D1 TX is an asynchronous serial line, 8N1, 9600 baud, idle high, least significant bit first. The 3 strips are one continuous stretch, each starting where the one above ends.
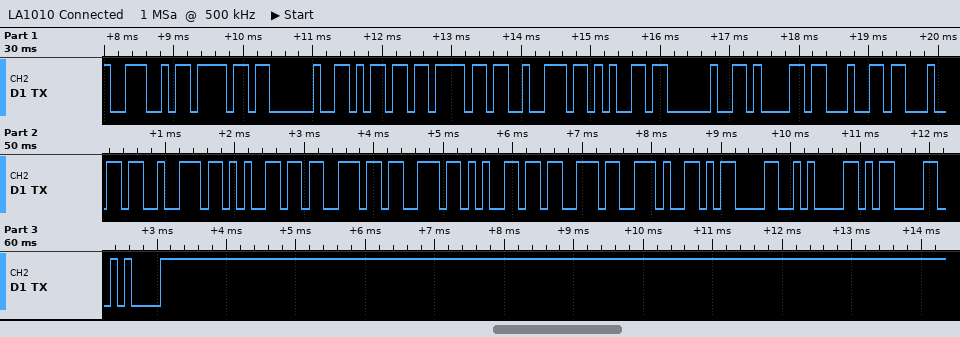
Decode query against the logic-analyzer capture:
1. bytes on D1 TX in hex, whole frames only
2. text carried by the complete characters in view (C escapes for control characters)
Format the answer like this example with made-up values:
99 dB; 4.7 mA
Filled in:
4E 6F 20 6D 6F 72 65 20 61 64 64 72 65 73 73 65 73 2E 0D 0A 0D 0A; "No more addresses.\r\n\r\n"
